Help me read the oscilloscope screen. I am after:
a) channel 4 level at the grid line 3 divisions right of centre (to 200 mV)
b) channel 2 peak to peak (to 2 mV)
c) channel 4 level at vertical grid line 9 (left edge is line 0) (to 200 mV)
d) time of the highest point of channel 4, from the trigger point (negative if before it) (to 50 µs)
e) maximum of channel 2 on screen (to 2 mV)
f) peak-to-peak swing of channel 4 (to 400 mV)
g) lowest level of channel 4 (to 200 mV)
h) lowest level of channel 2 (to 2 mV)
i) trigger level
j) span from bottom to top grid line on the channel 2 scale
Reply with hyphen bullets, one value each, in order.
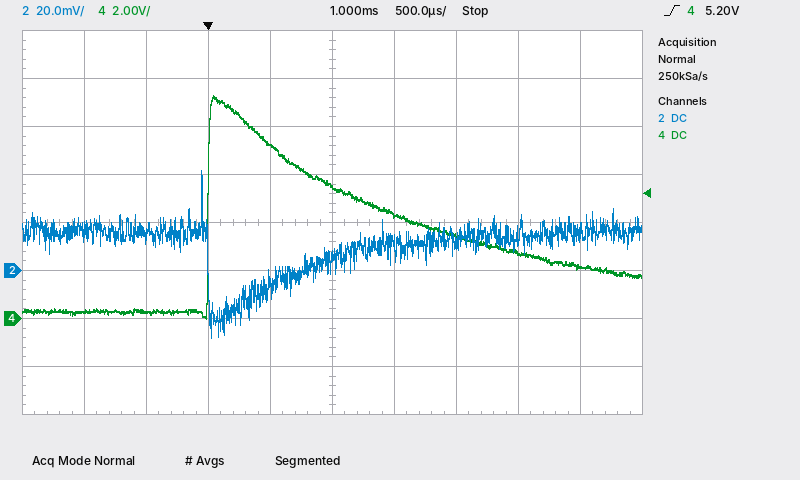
- 2.8 V
- 70 mV
- 2.2 V
- +50 µs
- 42 mV
- 9.2 V
- 0.0 V
- -28 mV
- 5.20 V
- 160 mV
